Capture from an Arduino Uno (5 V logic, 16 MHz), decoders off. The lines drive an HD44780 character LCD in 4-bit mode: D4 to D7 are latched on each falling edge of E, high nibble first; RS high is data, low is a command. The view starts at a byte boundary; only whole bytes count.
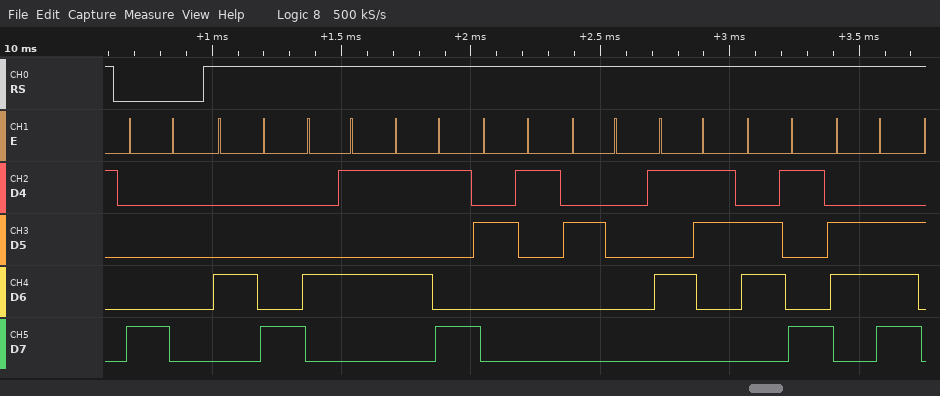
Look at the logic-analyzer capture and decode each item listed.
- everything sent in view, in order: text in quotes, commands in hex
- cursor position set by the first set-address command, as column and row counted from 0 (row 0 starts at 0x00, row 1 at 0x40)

0x80 "HEY! Sin"
column 0, row 0
